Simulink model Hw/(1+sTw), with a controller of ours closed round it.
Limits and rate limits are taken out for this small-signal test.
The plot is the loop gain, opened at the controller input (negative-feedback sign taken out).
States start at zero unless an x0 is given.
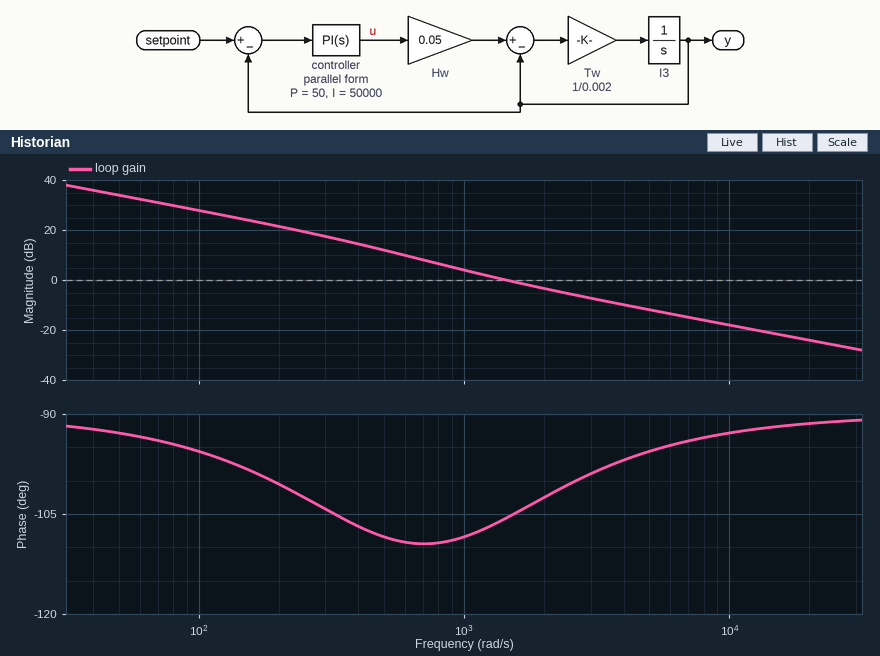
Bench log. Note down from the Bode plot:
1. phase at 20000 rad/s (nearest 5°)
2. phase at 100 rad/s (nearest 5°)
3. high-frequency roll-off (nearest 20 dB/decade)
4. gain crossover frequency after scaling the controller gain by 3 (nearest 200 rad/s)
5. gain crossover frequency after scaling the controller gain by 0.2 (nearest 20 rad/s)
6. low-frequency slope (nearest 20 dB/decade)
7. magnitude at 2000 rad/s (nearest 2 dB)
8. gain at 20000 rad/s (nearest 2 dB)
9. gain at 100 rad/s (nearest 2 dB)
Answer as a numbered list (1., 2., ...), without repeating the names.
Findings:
1. -90°
2. -95°
3. -20 dB/decade
4. 3800 rad/s
5. 420 rad/s
6. -20 dB/decade
7. -4 dB
8. -24 dB
9. 28 dB
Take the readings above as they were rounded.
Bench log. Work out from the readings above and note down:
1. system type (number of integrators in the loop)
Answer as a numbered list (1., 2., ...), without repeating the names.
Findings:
1. 1
